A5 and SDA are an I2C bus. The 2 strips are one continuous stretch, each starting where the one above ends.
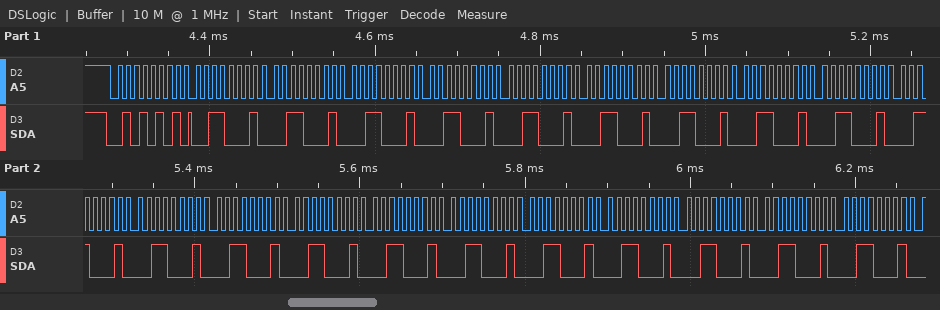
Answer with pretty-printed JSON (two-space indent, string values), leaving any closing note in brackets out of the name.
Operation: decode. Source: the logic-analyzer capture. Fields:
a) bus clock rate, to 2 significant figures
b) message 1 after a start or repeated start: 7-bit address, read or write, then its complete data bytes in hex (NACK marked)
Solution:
{
  "bus clock rate, to 2 significant figures": "100 kHz",
  "message 1 after a start or repeated start: 7-bit address, read or write, then its complete data bytes in hex": "0x2A read: 31 31 31 31 31 31 31 31 31 31 31 31 31 31 31 31 31 31 31 31"
}
